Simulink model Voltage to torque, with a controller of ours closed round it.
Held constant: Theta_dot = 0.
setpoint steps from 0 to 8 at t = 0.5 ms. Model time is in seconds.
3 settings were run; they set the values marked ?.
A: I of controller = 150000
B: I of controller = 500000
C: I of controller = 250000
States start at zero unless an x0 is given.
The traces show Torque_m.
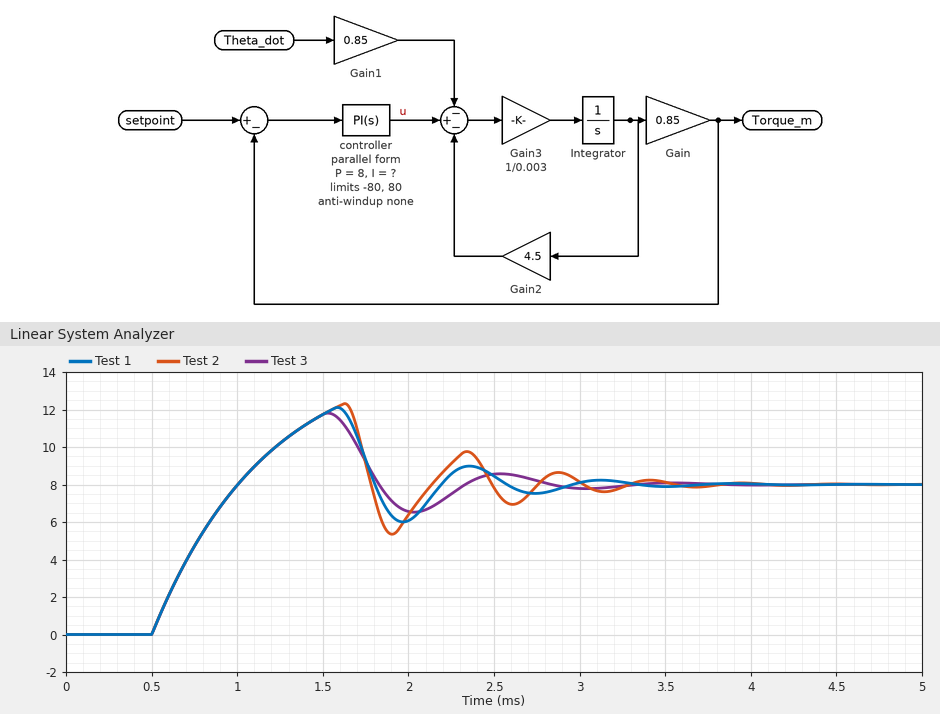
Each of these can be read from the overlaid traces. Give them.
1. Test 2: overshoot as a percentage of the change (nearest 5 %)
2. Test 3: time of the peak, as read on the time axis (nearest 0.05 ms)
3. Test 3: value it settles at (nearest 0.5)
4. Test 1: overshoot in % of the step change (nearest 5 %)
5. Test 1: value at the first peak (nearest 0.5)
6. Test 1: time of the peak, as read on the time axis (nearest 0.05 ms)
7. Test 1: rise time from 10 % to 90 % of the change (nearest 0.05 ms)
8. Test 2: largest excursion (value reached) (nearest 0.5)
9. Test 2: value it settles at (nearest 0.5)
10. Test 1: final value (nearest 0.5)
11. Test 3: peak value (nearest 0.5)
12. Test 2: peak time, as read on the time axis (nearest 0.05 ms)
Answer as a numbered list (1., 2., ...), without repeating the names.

1. 55 %
2. 1.55 ms
3. 8.0
4. 50 %
5. 12.0
6. 1.60 ms
7. 0.40 ms
8. 12.5
9. 8.0
10. 8.0
11. 12.0
12. 1.65 ms
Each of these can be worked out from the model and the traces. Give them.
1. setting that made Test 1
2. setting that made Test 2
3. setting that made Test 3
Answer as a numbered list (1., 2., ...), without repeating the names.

1. C
2. B
3. A
